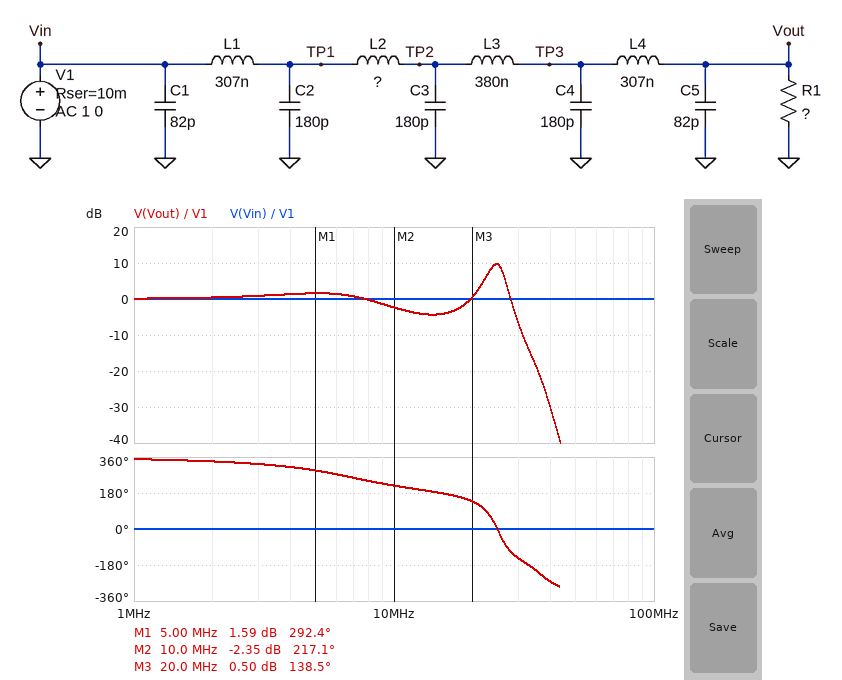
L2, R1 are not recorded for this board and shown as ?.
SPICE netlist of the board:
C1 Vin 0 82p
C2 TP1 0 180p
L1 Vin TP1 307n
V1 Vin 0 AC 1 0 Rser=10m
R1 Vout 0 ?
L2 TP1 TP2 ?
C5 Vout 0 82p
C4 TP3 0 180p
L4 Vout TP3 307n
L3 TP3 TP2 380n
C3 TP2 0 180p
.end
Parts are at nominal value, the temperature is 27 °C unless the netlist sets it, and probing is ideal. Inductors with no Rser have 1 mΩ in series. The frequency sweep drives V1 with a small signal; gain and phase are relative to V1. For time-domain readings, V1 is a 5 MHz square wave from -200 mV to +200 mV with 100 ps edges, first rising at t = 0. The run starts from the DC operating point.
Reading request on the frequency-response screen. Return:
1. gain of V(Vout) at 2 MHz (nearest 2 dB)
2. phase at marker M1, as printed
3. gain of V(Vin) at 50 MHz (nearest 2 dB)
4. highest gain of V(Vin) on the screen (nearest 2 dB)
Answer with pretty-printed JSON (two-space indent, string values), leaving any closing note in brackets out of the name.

{
  "gain of V(Vout) at 2 MHz": "0 dB",
  "phase at marker M1, as printed": "292.4 deg",
  "gain of V(Vin) at 50 MHz": "0 dB",
  "highest gain of V(Vin) on the screen": "0 dB"
}
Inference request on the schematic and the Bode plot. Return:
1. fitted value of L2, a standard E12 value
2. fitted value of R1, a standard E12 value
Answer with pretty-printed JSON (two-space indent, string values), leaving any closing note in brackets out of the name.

{
  "fitted value of L2, a standard E12 value": "1 µH",
  "fitted value of R1, a standard E12 value": "68 Ω"
}
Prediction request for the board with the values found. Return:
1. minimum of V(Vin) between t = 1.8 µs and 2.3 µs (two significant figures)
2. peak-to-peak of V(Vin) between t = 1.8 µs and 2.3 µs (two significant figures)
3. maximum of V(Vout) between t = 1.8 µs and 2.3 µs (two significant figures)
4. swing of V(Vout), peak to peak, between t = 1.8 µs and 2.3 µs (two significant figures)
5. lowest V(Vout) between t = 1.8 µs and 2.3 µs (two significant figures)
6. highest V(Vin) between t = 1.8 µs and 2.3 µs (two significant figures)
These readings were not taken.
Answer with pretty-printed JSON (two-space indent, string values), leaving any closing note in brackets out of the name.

{
  "minimum of V(Vin) between t = 1.8 µs and 2.3 µs": "-200 mV",
  "peak-to-peak of V(Vin) between t = 1.8 µs and 2.3 µs": "400 mV",
  "maximum of V(Vout) between t = 1.8 µs and 2.3 µs": "420 mV",
  "swing of V(Vout), peak to peak, between t = 1.8 µs and 2.3 µs": "840 mV",
  "lowest V(Vout) between t = 1.8 µs and 2.3 µs": "-420 mV",
  "highest V(Vin) between t = 1.8 µs and 2.3 µs": "200 mV"
}
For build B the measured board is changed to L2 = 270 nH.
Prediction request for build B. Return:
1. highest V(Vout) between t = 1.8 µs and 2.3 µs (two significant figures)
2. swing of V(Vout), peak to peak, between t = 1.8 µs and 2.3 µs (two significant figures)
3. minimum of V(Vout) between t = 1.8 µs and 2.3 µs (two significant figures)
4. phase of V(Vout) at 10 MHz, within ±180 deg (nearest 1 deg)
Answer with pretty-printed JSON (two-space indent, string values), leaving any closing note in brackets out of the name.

{
  "highest V(Vout) between t = 1.8 µs and 2.3 µs": "380 mV",
  "swing of V(Vout), peak to peak, between t = 1.8 µs and 2.3 µs": "760 mV",
  "minimum of V(Vout) between t = 1.8 µs and 2.3 µs": "-380 mV",
  "phase of V(Vout) at 10 MHz, within ±180 deg": "-115 deg"
}
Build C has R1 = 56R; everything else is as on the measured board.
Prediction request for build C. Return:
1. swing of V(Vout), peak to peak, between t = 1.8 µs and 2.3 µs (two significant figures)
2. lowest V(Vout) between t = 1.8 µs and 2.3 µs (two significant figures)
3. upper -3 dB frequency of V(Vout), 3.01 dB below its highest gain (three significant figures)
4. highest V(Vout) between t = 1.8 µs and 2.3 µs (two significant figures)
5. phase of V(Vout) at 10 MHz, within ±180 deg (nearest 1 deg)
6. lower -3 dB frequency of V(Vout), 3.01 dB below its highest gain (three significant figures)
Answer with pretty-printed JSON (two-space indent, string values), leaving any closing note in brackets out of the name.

{
  "swing of V(Vout), peak to peak, between t = 1.8 µs and 2.3 µs": "740 mV",
  "lowest V(Vout) between t = 1.8 µs and 2.3 µs": "-370 mV",
  "upper -3 dB frequency of V(Vout), 3.01 dB below its highest gain": "26.1 MHz",
  "highest V(Vout) between t = 1.8 µs and 2.3 µs": "370 mV",
  "phase of V(Vout) at 10 MHz, within ±180 deg": "-137 deg",
  "lower -3 dB frequency of V(Vout), 3.01 dB below its highest gain": "23.5 MHz"
}
